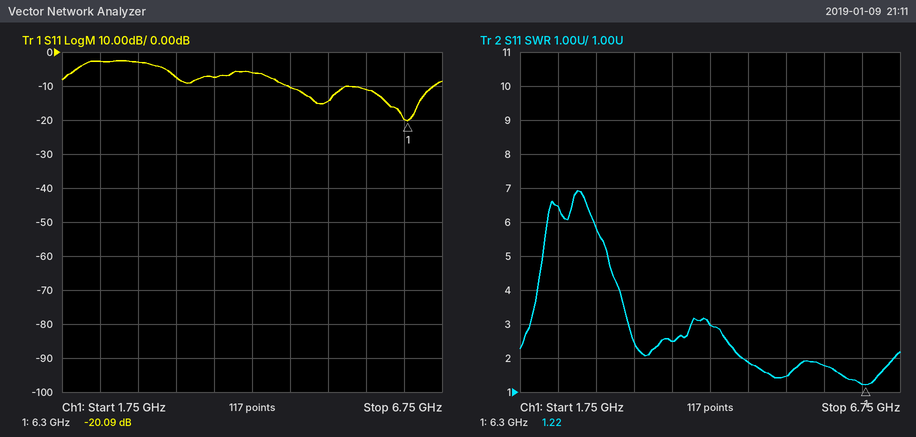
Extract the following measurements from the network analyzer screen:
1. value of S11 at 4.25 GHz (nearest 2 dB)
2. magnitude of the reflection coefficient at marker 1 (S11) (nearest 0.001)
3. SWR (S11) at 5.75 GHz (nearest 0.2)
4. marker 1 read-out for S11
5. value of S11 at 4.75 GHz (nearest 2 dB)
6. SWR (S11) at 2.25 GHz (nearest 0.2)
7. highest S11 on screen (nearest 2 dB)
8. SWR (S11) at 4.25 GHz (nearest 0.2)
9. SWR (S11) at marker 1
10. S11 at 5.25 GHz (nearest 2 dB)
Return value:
-6 dB
0.099
1.8
-20.09 dB
-10 dB
6.4
-2 dB
3.0
1.22
-14 dB
